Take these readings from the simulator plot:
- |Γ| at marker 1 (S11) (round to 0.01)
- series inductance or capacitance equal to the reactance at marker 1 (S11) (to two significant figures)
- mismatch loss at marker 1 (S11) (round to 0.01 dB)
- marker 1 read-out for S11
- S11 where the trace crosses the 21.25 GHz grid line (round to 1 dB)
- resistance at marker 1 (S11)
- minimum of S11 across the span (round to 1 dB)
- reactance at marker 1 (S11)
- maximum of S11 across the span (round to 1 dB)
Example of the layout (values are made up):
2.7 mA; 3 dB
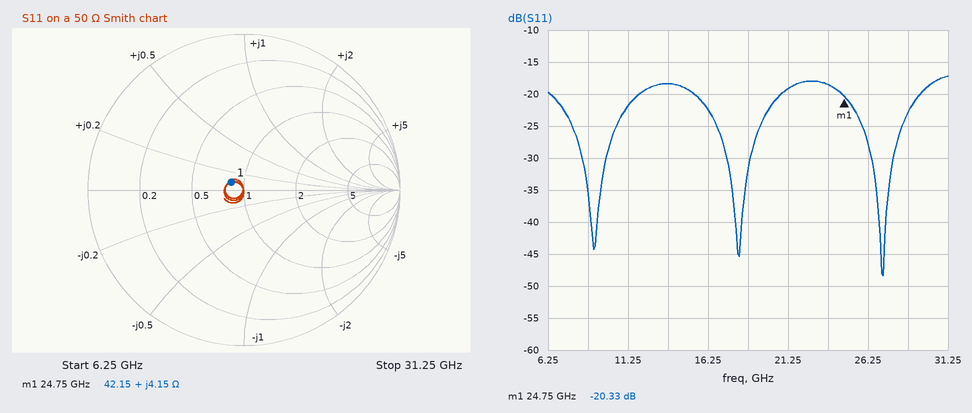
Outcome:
0.10; 27 pH; 0.04 dB; -20.33 dB; -19 dB; 42.15 Ω; -48 dB; +4.15 Ω; -17 dB
